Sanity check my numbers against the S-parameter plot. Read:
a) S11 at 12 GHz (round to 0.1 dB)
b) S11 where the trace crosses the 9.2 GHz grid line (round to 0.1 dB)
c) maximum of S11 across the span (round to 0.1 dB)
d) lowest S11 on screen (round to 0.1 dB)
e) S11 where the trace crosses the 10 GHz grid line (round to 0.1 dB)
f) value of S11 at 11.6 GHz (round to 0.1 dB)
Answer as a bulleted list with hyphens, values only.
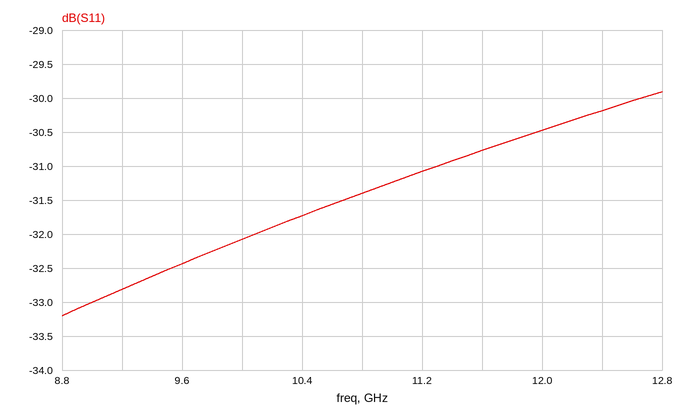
- -30.5 dB
- -32.8 dB
- -29.9 dB
- -33.2 dB
- -32.1 dB
- -30.8 dB
